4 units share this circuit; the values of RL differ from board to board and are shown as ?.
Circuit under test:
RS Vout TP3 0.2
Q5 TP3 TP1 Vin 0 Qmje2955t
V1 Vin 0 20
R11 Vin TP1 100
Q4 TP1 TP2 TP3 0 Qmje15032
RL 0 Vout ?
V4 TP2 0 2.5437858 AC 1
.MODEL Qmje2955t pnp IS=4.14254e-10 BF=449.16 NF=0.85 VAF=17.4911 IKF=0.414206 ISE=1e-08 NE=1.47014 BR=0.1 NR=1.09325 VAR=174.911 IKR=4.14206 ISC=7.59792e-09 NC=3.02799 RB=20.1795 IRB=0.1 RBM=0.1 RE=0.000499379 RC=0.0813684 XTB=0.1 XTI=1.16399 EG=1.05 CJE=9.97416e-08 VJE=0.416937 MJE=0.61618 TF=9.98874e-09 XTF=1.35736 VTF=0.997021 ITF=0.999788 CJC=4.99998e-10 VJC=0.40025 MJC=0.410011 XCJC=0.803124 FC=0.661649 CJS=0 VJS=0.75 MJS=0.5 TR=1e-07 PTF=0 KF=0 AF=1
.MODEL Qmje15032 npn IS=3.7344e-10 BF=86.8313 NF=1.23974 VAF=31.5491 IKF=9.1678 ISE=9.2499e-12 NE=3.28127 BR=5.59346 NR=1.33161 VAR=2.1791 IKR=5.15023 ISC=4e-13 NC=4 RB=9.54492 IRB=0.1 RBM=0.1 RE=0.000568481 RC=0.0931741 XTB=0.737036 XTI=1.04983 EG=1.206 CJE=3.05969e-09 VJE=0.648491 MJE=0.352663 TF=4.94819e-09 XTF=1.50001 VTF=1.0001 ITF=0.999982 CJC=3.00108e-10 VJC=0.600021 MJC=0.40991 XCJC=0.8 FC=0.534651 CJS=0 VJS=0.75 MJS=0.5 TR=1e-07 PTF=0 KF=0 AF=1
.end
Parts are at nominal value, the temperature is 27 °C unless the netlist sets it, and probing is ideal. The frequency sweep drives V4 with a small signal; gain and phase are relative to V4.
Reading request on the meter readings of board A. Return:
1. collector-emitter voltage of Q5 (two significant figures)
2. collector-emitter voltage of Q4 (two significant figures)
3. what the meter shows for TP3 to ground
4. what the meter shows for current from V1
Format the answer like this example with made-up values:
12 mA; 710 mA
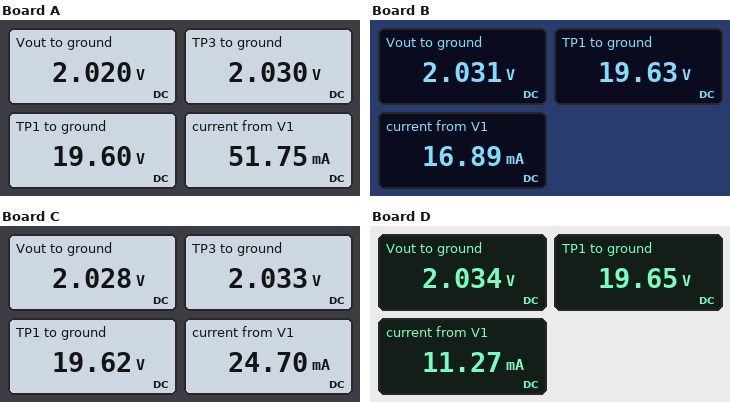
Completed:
-18 V; 18 V; 2.030 V; 51.75 mA
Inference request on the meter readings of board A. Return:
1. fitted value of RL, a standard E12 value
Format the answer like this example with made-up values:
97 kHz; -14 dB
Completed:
39 Ω
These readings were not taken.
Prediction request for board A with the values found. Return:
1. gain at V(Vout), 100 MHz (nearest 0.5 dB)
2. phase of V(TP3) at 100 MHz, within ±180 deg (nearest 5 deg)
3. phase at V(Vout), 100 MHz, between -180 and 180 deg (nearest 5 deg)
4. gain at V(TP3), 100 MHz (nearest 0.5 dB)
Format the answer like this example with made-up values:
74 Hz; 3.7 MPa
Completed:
-5.0 dB; -25 deg; -25 deg; -5.0 dB
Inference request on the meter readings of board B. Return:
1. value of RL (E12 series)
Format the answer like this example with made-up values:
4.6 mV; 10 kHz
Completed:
120 Ω
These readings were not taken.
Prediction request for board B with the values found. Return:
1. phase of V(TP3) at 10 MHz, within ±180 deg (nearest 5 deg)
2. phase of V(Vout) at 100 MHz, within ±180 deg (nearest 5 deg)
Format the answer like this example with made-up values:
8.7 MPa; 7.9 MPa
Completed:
-5 deg; -30 deg
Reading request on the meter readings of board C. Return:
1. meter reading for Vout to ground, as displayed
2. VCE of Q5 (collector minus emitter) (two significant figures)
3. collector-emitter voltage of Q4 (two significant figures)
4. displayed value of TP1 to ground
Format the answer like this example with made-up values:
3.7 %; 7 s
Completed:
2.028 V; -18 V; 18 V; 19.62 V
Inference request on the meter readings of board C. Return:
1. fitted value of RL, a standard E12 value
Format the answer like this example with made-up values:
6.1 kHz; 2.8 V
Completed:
82 Ω
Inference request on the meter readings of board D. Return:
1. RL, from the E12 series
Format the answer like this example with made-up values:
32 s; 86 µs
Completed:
180 Ω
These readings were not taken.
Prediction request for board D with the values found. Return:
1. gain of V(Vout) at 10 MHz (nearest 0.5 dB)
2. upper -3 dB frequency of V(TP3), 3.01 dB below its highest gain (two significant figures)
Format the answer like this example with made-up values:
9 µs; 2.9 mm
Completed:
-0.5 dB; 76 MHz
